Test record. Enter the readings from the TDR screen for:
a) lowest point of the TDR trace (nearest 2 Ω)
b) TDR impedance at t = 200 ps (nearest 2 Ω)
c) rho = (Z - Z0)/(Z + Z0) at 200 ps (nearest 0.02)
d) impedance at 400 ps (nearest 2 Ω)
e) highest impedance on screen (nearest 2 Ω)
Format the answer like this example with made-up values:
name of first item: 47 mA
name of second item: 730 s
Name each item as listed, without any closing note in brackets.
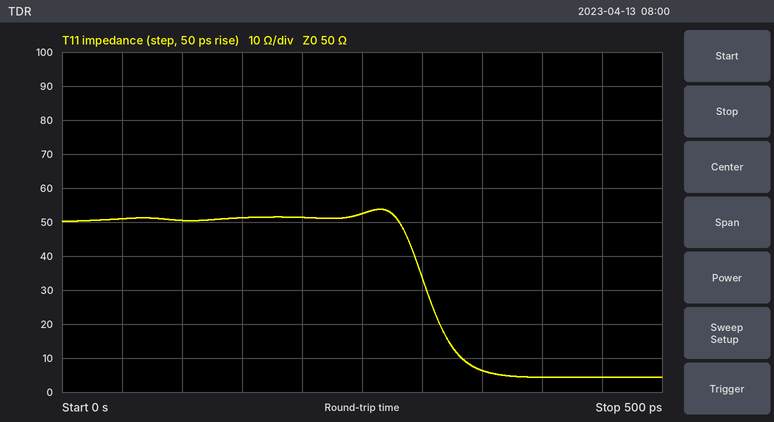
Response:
lowest point of the TDR trace: 4 Ω
TDR impedance at t = 200 ps: 52 Ω
rho = (Z - Z0)/(Z + Z0) at 200 ps: +0.02
impedance at 400 ps: 4 Ω
highest impedance on screen: 54 Ω
